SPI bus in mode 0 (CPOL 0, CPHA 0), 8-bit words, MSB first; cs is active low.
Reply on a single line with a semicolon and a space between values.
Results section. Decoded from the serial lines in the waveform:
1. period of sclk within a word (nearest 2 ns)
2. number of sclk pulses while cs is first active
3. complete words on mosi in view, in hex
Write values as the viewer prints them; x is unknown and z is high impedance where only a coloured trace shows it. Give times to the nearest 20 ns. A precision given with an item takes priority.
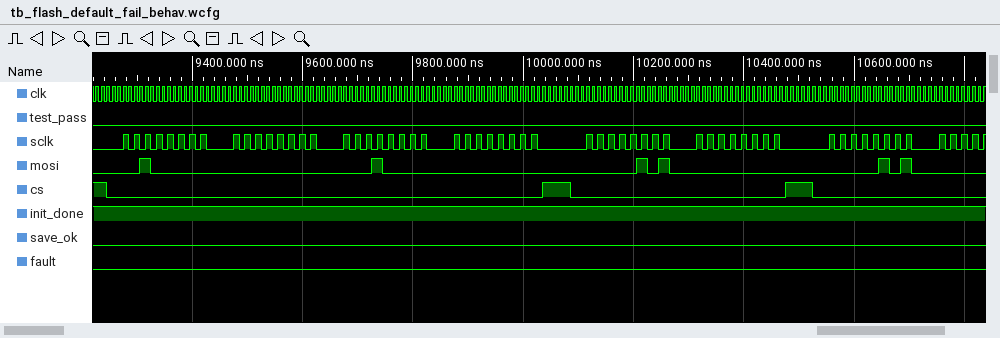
20 ns; 32; 20, 00, 10, 00, 05, 00, 05
